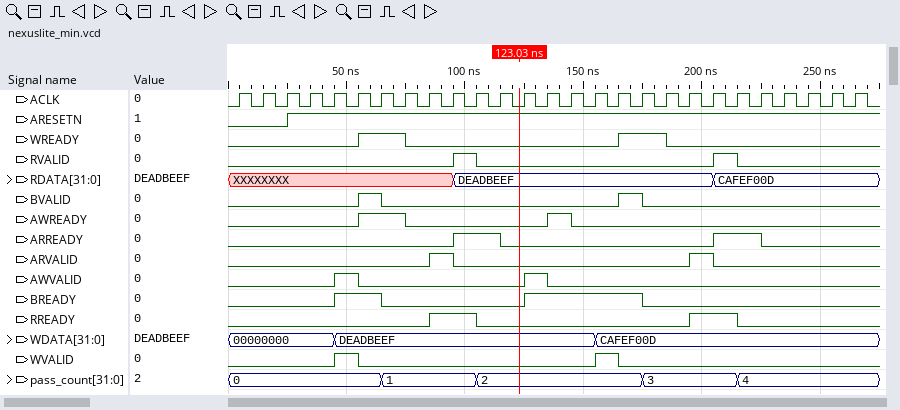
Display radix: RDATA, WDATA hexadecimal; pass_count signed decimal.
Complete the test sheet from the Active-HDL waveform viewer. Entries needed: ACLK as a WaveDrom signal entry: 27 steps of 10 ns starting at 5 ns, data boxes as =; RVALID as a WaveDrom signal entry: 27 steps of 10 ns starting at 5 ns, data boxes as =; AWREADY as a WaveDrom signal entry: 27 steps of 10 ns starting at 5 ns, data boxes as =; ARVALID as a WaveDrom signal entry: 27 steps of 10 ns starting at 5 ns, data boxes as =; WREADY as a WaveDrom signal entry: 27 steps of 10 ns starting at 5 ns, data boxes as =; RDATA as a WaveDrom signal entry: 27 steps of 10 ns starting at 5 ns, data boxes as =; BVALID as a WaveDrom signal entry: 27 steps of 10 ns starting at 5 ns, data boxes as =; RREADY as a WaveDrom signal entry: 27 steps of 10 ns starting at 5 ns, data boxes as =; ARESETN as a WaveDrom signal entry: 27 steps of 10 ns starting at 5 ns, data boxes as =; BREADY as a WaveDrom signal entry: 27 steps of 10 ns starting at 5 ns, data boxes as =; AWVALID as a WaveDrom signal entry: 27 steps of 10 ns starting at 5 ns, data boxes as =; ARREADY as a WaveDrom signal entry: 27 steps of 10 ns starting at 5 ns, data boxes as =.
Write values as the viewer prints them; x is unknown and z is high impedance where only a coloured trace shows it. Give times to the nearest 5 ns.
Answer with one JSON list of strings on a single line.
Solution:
["{name: 'ACLK', wave: 'p..........................'}", "{name: 'RVALID', wave: '0........10.........10.....'}", "{name: 'AWREADY', wave: '0....1.0.....10............'}", "{name: 'ARVALID', wave: '0.......10.........10......'}", "{name: 'WREADY', wave: '0....1.0........1.0........'}", "{name: 'RDATA', wave: 'x........=..........=......', data: 'DEADBEEF CAFEF00D'}", "{name: 'BVALID', wave: '0....10.........10.........'}", "{name: 'RREADY', wave: '0.......1.0........1.0.....'}", "{name: 'ARESETN', wave: '0.1........................'}", "{name: 'BREADY', wave: '0...1.0.....1....0.........'}", "{name: 'AWVALID', wave: '0...10......10.............'}", "{name: 'ARREADY', wave: '0........1.0........1.0....'}"]
